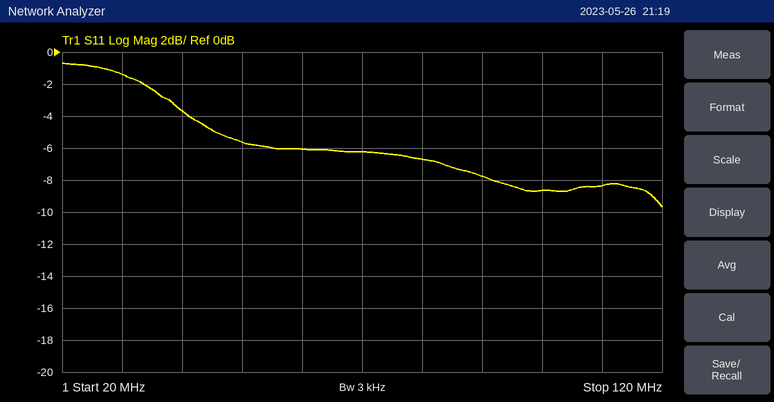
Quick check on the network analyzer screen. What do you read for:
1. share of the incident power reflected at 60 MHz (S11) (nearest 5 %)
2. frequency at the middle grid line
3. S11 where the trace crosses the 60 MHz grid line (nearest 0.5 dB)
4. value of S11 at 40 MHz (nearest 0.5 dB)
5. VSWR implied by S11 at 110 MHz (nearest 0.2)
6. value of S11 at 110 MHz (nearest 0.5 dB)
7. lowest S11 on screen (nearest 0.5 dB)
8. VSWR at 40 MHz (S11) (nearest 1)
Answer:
25 %
70 MHz
-6.0 dB
-3.5 dB
2.2
-8.5 dB
-9.5 dB
5
